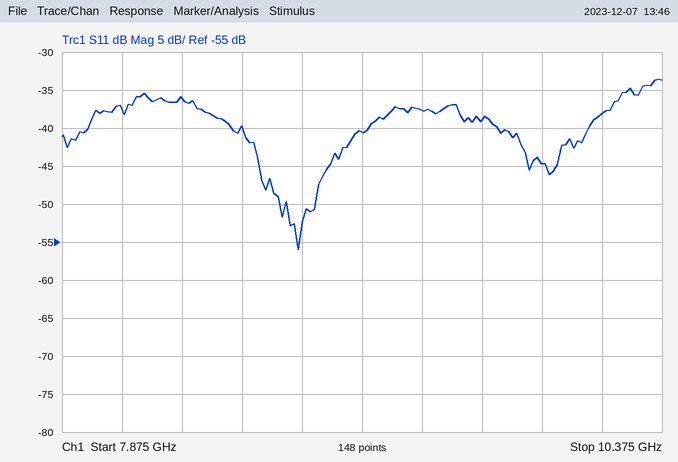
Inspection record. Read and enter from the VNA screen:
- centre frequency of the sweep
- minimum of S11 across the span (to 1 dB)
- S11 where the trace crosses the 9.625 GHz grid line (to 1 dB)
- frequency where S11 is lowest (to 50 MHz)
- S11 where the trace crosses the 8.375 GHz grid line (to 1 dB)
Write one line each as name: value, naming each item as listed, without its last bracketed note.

centre frequency of the sweep: 9.125 GHz
minimum of S11 across the span: -56 dB
S11 where the trace crosses the 9.625 GHz grid line: -39 dB
frequency where S11 is lowest: 8.85 GHz
S11 where the trace crosses the 8.375 GHz grid line: -36 dB
